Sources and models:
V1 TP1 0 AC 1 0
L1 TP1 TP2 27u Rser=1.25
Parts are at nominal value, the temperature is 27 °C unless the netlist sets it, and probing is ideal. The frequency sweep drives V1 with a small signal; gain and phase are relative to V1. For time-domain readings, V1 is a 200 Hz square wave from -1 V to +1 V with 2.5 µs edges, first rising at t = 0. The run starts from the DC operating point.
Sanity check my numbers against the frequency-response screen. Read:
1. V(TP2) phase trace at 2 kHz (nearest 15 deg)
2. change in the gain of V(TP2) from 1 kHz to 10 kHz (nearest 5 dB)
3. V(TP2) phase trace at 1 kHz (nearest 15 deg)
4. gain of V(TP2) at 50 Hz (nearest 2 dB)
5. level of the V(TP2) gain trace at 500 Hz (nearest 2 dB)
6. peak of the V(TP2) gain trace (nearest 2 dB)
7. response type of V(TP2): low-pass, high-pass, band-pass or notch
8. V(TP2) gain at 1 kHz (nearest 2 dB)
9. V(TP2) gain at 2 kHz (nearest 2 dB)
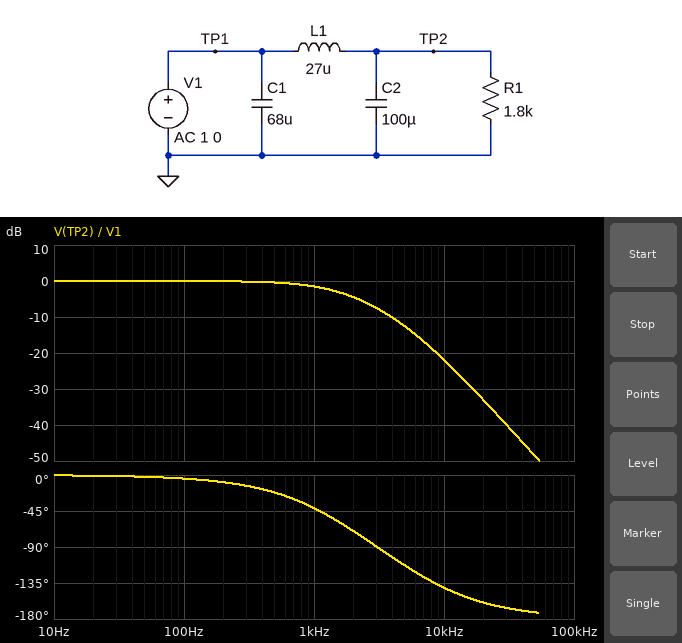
-75 deg
-20 dB
-45 deg
0 dB
0 dB
0 dB
low-pass
-2 dB
-4 dB
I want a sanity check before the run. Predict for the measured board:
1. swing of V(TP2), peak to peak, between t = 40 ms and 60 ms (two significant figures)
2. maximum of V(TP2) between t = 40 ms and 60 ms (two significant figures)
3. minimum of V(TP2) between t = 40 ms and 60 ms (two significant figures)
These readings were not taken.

2.0 V
1.0 V
-1.0 V
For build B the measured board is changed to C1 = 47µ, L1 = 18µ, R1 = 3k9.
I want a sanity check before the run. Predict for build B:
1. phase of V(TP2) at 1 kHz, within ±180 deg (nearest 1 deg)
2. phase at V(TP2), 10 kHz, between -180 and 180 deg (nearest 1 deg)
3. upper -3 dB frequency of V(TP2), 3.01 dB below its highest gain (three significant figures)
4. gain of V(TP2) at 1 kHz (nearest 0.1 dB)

-40 deg
-128 deg
1.44 kHz
-1.7 dB
